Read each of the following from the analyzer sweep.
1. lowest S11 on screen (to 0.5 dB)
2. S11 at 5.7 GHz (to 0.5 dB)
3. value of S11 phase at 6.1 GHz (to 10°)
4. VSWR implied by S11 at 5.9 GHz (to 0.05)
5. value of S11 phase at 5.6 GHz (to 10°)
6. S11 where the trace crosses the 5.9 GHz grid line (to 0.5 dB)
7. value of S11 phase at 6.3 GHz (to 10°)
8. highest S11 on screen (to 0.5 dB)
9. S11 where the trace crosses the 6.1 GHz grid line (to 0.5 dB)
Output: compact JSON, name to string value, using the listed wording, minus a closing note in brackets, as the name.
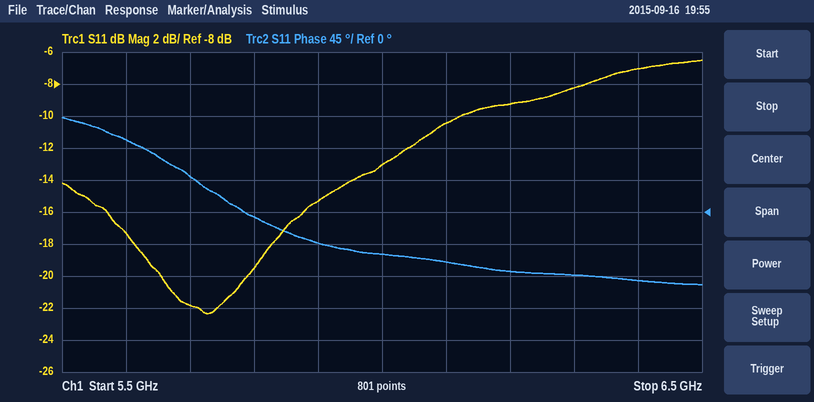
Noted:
{"lowest S11 on screen": "-22.5 dB", "S11 at 5.7 GHz": "-22.0 dB", "value of S11 phase at 6.1 GHz": "-70°", "VSWR implied by S11 at 5.9 GHz": "1.40", "value of S11 phase at 5.6 GHz": "100°", "S11 where the trace crosses the 5.9 GHz grid line": "-15.5 dB", "value of S11 phase at 6.3 GHz": "-90°", "highest S11 on screen": "-6.5 dB", "S11 where the trace crosses the 6.1 GHz grid line": "-10.5 dB"}
